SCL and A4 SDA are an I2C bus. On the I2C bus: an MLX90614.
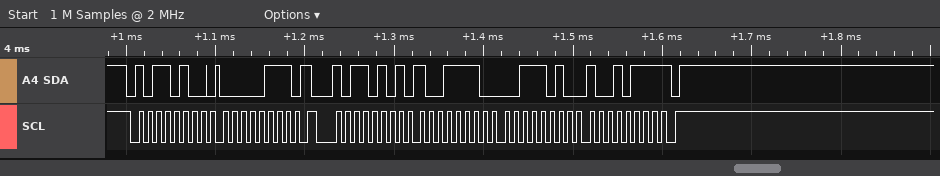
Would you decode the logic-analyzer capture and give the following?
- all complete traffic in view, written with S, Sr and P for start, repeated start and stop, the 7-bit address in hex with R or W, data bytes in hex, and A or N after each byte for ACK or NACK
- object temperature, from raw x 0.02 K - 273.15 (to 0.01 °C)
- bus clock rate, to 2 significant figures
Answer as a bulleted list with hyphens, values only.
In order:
- S 5AW A 07 A Sr 5AR A 9E A 3A A 97 N P
- 26.97 °C
- 100 kHz
